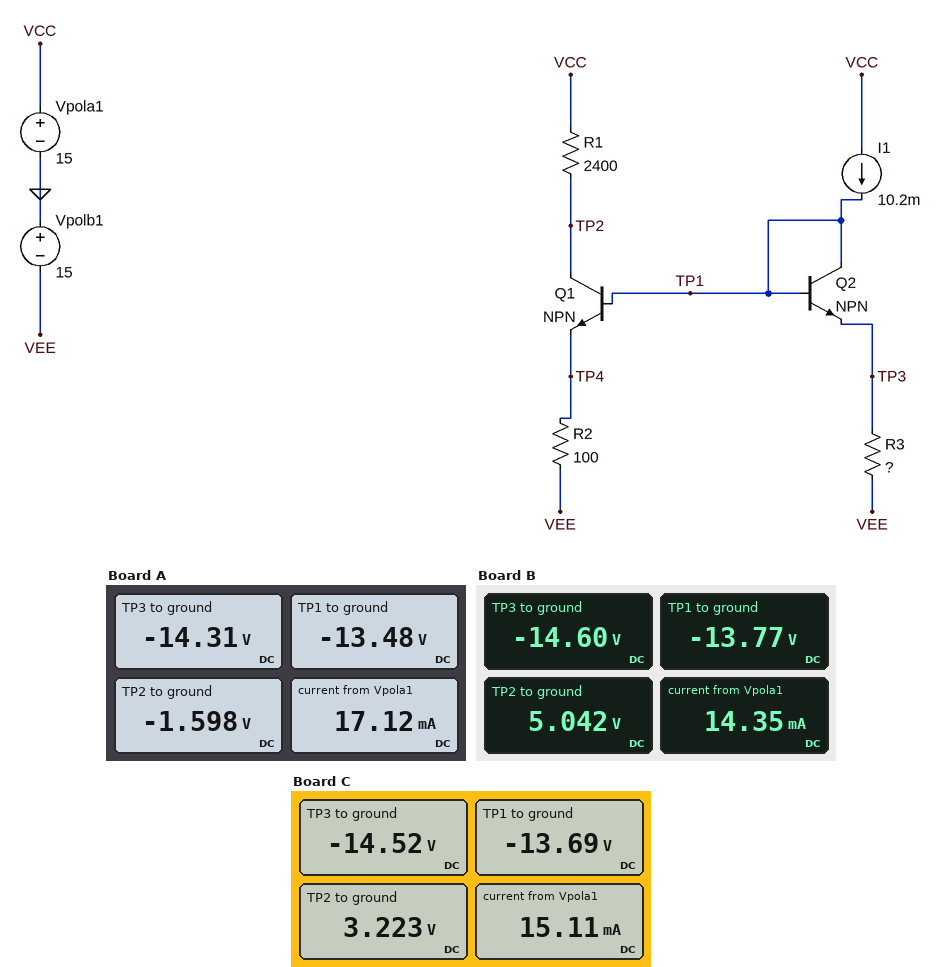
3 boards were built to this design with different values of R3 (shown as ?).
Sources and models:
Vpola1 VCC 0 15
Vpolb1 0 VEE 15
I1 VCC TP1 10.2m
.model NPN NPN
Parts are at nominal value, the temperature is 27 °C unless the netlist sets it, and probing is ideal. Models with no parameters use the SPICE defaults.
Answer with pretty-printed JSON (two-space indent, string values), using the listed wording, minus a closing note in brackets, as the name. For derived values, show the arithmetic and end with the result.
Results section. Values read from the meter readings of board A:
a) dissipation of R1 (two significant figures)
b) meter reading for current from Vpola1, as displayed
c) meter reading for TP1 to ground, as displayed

{
  "dissipation of R1": "(15 V - (-1.598 V))^2 / 2.4 kΩ = 110 mW",
  "meter reading for current from Vpola1, as displayed": "17.12 mA",
  "meter reading for TP1 to ground, as displayed": "-13.48 V"
}
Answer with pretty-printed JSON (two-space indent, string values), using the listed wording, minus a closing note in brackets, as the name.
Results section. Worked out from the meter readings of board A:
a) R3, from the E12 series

{
  "R3, from the E12 series": "68 Ω"
}
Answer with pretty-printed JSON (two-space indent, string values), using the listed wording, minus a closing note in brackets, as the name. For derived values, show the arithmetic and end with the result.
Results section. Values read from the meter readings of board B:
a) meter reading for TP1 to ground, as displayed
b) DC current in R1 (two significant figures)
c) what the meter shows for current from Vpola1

{
  "meter reading for TP1 to ground, as displayed": "-13.77 V",
  "DC current in R1": "(15 V - 5.042 V) / 2.4 kΩ = 4.1 mA",
  "what the meter shows for current from Vpola1": "14.35 mA"
}
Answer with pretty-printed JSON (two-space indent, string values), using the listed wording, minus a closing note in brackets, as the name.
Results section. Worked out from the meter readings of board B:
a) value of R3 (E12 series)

{
  "value of R3": "39 Ω"
}
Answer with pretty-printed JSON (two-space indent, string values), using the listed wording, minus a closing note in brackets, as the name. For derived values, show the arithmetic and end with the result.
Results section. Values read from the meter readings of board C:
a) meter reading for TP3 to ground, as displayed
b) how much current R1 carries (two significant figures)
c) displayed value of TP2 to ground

{
  "meter reading for TP3 to ground, as displayed": "-14.52 V",
  "how much current R1 carries": "(15 V - 3.223 V) / 2.4 kΩ = 4.9 mA",
  "displayed value of TP2 to ground": "3.223 V"
}
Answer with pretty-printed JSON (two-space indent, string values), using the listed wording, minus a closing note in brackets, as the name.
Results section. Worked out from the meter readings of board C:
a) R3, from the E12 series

{
  "R3, from the E12 series": "47 Ω"
}
